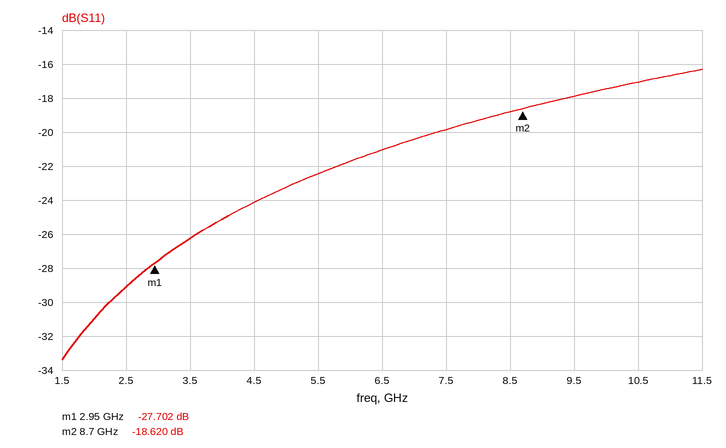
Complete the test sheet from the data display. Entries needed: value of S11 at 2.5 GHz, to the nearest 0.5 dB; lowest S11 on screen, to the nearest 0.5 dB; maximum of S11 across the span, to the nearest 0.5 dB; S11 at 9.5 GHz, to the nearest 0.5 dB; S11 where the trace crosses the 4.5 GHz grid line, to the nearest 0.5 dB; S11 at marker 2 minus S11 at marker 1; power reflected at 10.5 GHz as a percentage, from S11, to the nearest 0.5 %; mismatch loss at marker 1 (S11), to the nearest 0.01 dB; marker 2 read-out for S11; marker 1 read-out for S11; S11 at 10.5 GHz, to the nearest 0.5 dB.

-29.0 dB
-33.5 dB
-16.5 dB
-18.0 dB
-24.0 dB
9.082 dB
2.0 %
0.01 dB
-18.620 dB
-27.702 dB
-17.0 dB
